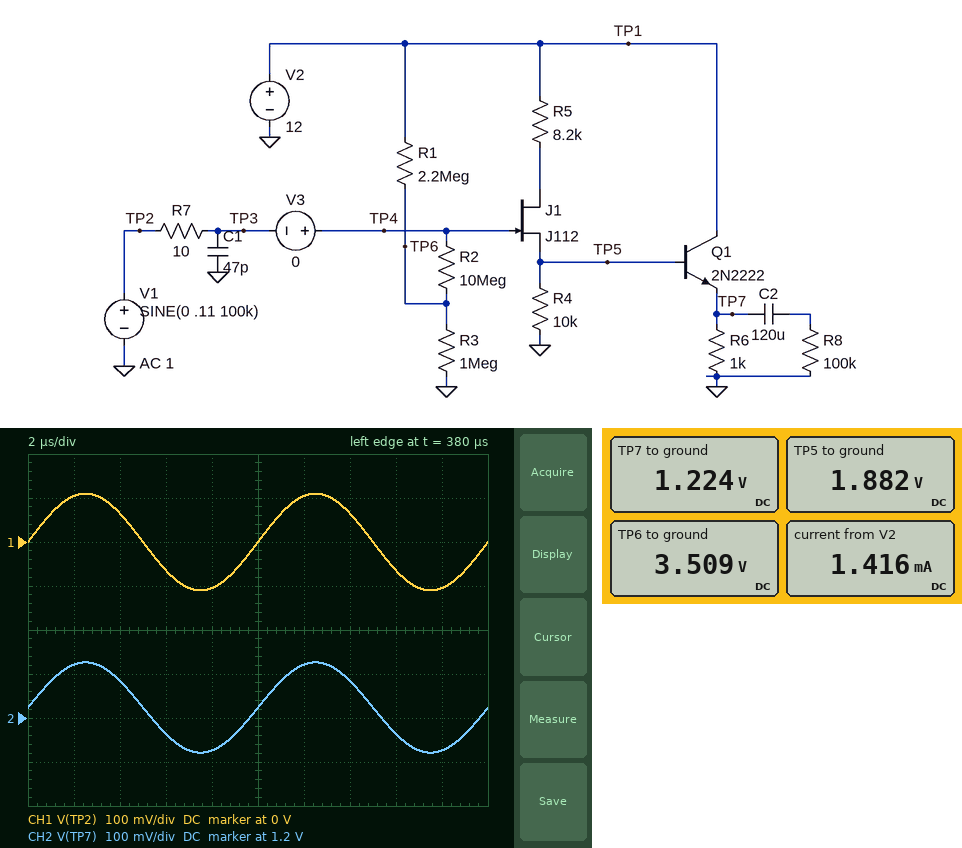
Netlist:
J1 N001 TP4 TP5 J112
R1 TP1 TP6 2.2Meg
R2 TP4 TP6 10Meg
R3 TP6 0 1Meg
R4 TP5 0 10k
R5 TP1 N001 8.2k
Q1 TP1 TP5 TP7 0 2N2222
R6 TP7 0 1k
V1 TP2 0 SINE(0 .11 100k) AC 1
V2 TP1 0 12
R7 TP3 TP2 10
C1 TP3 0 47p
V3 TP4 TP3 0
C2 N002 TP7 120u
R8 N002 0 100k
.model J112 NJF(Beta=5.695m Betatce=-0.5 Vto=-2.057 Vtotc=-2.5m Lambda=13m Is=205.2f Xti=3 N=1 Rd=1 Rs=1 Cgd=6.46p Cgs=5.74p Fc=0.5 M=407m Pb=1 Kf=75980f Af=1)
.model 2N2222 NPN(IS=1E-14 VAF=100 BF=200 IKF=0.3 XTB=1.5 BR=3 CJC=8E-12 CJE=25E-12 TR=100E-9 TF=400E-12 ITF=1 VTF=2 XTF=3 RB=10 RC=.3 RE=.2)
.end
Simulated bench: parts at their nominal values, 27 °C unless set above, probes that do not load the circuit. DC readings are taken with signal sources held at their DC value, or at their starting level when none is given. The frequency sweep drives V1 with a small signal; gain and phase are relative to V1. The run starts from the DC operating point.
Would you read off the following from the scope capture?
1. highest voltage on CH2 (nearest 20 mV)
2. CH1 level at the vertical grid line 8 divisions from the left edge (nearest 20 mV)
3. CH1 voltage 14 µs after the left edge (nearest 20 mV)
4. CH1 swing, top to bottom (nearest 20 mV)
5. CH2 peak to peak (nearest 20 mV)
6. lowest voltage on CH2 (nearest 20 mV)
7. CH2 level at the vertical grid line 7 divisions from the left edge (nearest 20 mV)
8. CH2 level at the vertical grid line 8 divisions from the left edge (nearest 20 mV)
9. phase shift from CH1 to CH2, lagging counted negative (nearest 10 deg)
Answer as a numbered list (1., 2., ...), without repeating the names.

1. 1.32 V
2. -60 mV
3. 60 mV
4. 220 mV
5. 200 mV
6. 1.12 V
7. 1.28 V
8. 1.16 V
9. 0 deg
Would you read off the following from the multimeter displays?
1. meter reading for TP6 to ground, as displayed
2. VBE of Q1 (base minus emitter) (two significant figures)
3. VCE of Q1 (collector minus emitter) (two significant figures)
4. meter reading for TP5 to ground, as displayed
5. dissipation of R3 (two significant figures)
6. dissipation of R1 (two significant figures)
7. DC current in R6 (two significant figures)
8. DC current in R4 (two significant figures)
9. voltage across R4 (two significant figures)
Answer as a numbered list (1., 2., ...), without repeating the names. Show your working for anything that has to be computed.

1. 3.509 V
2. 1.882 V - 1.224 V = 660 mV
3. 12 V - 1.224 V = 11 V
4. 1.882 V
5. (3.509 V)^2 / 1 MΩ = 12 µW
6. (12 V - 3.509 V)^2 / 2.2 MΩ = 33 µW
7. (1.224 V) / 1 kΩ = 1.2 mA
8. (1.882 V) / 10 kΩ = 190 µA
9. 1.882 V = 1.9 V
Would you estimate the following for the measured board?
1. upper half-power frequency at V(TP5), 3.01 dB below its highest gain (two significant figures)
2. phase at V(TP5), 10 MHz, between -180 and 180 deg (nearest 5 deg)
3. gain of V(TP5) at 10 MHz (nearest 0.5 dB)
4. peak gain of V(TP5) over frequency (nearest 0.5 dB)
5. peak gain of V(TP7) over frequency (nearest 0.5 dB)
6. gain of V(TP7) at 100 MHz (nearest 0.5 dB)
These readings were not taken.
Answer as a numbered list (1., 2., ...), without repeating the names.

1. 55 MHz
2. -10 deg
3. -0.5 dB
4. -0.5 dB
5. -0.5 dB
6. -5.5 dB
